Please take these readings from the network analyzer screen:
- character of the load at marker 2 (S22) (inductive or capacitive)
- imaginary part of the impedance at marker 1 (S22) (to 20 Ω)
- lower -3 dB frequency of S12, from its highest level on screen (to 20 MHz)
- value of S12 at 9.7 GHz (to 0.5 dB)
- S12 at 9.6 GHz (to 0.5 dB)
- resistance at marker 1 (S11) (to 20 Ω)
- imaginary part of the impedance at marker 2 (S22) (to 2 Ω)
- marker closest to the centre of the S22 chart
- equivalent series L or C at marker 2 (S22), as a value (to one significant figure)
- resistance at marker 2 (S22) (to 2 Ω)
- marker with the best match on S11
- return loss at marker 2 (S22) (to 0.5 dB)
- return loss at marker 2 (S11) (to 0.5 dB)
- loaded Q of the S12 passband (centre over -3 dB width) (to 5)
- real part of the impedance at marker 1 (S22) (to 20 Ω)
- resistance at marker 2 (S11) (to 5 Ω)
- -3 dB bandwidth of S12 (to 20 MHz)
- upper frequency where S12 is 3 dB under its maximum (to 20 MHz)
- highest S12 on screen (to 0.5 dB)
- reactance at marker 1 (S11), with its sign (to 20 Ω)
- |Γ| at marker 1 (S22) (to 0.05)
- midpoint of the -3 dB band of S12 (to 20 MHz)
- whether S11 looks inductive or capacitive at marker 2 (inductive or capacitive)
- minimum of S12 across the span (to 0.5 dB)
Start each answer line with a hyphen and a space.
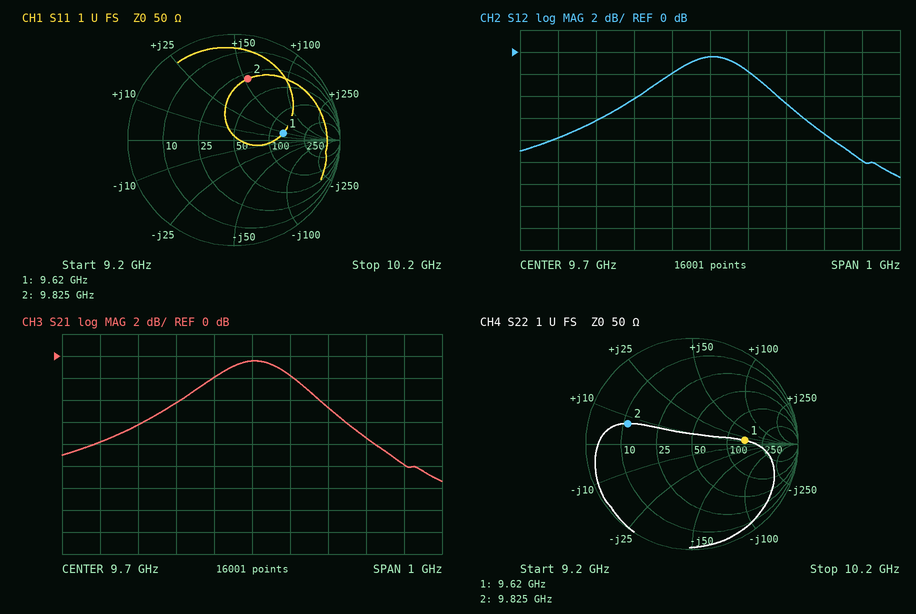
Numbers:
- inductive
- +20 Ω
- 9.54 GHz
- -0.5 dB
- -2.0 dB
- 140 Ω
- +8 Ω
- marker 1
- 100 pH
- 12 Ω
- marker 1
- 4.0 dB
- 4.5 dB
- 30
- 140 Ω
- 30 Ω
- 320 MHz
- 9.86 GHz
- -0.5 dB
- +20 Ω
- 0.50
- 9.70 GHz
- inductive
- -11.5 dB
